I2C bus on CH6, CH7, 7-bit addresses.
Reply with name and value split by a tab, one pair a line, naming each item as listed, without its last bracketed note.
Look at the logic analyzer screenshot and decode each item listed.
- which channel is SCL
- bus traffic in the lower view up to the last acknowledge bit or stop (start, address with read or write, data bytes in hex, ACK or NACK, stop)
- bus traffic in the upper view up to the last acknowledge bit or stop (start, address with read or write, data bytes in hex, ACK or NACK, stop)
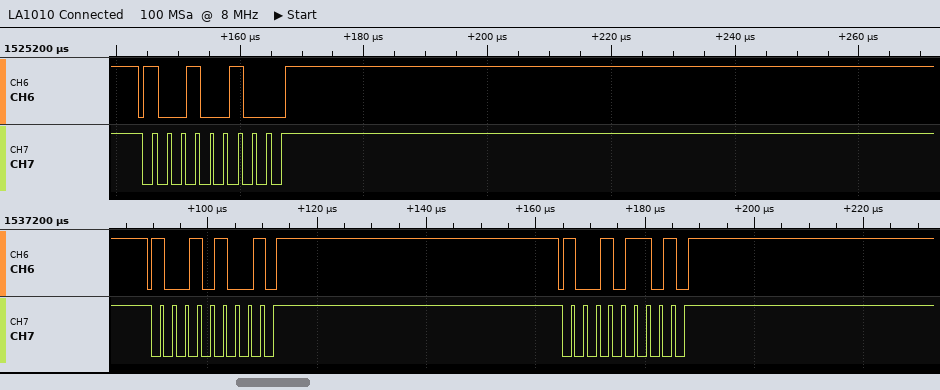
which channel is SCL	CH7
bus traffic in the lower view up to the last acknowledge bit or stop	start, address 4A write NACK, stop, start, address 4B write NACK, stop
bus traffic in the upper view up to the last acknowledge bit or stop	start, address 49 write ACK, stop
